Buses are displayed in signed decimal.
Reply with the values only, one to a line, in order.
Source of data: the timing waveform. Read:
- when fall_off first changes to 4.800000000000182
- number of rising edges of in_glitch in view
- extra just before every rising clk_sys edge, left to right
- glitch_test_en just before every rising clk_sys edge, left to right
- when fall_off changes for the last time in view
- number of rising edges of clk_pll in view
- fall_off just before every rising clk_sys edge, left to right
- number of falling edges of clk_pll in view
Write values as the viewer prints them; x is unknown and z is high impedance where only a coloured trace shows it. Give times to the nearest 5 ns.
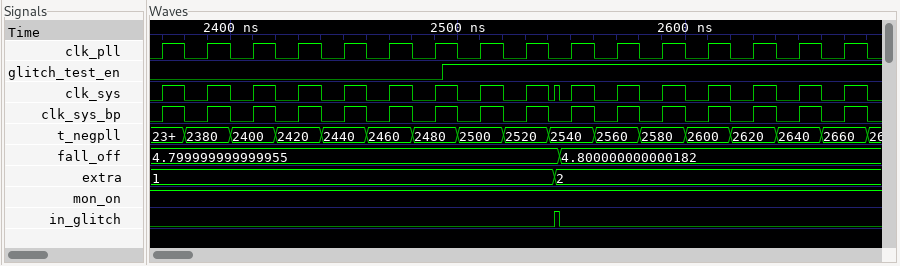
2545 ns
1
1, 1, 1, 1, 1, 1, 1, 1, 1, 1, 2, 2, 2, 2, 2, 2, 2
0 0 0 0 0 0 0 1 1 1 1 1 1 1 1 1 1
2545 ns
16
4.799999999999955, 4.799999999999955, 4.799999999999955, 4.799999999999955, 4.799999999999955, 4.799999999999955, 4.799999999999955, 4.799999999999955, 4.799999999999955, 4.799999999999955, 4.800000000000182, 4.800000000000182, 4.800000000000182, 4.800000000000182, 4.800000000000182, 4.800000000000182, 4.800000000000182
16
